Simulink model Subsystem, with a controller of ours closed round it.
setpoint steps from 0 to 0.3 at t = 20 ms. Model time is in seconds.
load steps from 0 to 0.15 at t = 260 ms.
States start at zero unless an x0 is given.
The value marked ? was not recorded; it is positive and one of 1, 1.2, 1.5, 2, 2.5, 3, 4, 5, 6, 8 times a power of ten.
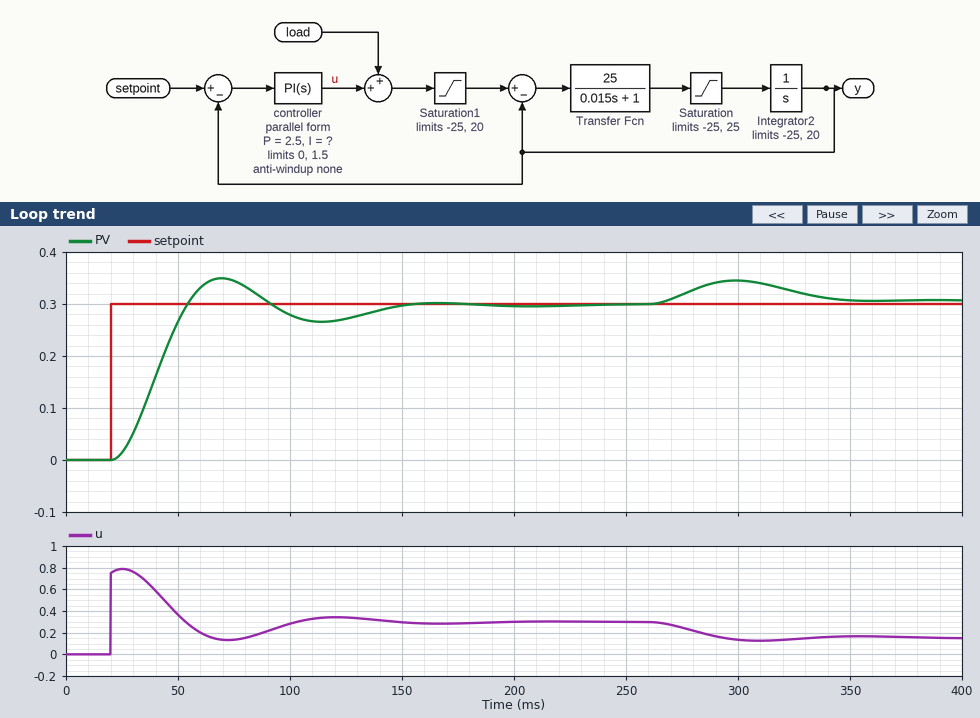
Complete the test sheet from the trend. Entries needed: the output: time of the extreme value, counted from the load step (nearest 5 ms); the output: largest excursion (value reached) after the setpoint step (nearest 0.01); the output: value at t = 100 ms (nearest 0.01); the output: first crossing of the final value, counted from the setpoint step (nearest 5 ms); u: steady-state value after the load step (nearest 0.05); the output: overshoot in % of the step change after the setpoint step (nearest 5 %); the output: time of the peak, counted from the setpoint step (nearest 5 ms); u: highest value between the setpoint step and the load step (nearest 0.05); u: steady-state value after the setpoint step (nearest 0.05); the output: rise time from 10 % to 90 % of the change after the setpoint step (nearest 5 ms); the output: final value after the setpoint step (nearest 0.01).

40 ms
0.35
0.28
35 ms
0.15
15 %
50 ms
0.80
0.30
25 ms
0.30
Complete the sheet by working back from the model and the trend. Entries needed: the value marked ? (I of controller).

50
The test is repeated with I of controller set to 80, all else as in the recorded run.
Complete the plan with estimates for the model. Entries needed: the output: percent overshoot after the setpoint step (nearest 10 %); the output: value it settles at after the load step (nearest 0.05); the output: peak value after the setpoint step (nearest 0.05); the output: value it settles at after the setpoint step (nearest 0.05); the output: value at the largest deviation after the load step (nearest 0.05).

30 %
0.30
0.40
0.30
0.35
